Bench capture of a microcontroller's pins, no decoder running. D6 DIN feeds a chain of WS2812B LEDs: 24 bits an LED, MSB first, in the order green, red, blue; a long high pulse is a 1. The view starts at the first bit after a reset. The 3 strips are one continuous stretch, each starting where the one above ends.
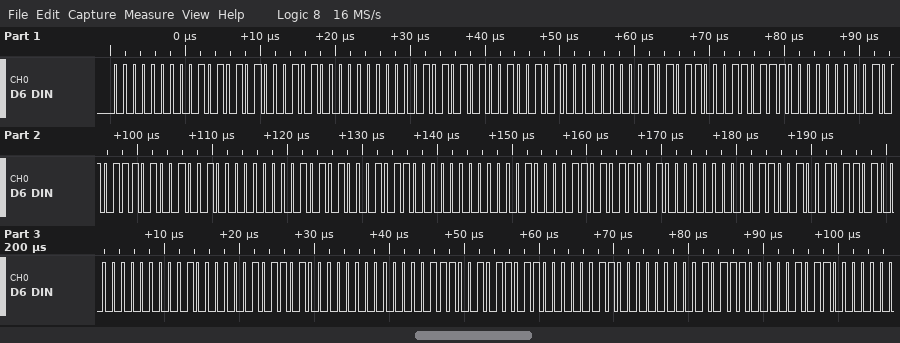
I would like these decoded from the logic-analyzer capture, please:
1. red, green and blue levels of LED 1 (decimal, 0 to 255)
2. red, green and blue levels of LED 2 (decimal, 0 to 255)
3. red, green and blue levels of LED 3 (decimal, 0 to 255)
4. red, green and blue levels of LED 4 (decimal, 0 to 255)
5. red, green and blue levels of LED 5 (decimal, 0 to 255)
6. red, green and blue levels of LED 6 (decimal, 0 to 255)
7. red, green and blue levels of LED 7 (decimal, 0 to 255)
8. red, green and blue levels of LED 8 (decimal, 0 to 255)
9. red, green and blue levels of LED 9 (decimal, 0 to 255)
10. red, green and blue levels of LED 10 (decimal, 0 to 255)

85, 0, 20
85, 0, 37
86, 0, 55
87, 0, 73
84, 0, 88
67, 0, 89
50, 0, 90
32, 0, 90
14, 0, 91
0, 3, 92
